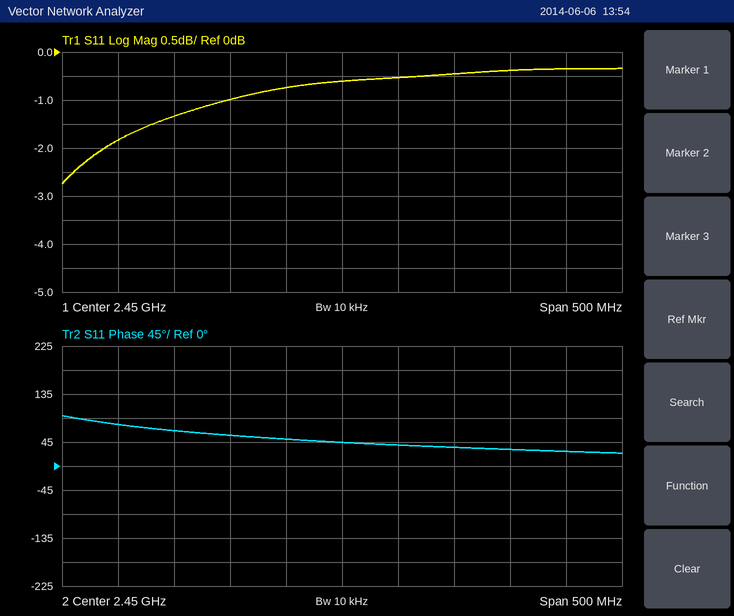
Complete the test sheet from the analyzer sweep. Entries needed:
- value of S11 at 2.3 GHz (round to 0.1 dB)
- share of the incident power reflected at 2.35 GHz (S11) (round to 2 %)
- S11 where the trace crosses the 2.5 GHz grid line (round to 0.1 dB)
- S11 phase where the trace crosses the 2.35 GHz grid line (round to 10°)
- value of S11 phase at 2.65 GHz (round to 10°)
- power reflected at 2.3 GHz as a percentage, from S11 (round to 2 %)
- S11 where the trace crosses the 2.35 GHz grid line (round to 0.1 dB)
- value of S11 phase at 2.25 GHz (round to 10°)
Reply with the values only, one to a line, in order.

-1.3 dB
80 %
-0.5 dB
60°
30°
74 %
-1.0 dB
80°
